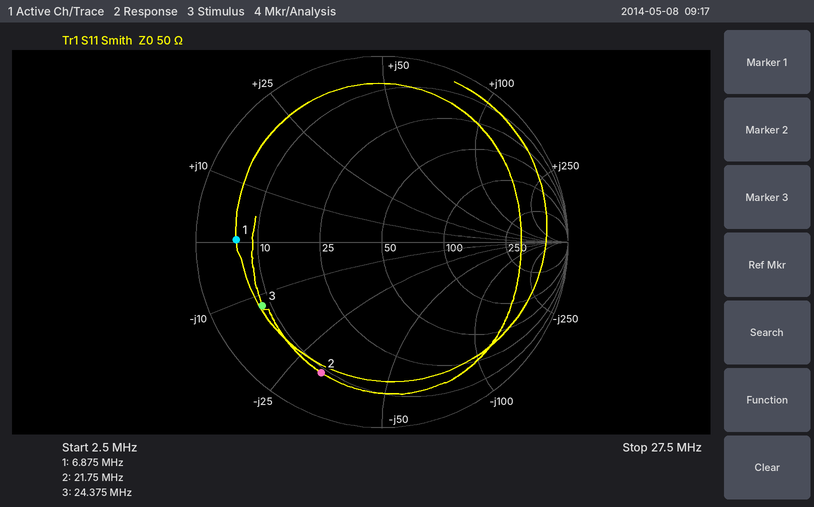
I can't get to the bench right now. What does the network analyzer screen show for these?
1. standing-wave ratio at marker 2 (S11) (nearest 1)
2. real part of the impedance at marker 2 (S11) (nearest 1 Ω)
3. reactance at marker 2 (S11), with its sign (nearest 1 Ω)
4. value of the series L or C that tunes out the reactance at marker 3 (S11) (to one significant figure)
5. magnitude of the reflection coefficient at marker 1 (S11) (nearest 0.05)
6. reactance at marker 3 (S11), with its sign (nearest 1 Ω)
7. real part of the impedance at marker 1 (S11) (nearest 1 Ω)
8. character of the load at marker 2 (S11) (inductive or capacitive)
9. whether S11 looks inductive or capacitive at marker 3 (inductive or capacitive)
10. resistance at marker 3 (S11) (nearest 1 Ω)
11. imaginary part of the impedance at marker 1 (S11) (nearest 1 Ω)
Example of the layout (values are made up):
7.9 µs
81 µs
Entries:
8
9 Ω
-31 Ω
80 nH
0.80
-12 Ω
6 Ω
capacitive
capacitive
8 Ω
0 Ω
